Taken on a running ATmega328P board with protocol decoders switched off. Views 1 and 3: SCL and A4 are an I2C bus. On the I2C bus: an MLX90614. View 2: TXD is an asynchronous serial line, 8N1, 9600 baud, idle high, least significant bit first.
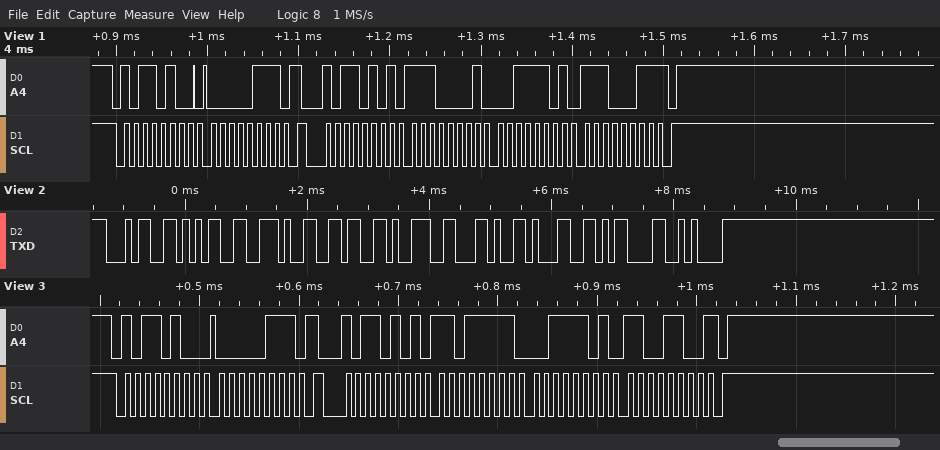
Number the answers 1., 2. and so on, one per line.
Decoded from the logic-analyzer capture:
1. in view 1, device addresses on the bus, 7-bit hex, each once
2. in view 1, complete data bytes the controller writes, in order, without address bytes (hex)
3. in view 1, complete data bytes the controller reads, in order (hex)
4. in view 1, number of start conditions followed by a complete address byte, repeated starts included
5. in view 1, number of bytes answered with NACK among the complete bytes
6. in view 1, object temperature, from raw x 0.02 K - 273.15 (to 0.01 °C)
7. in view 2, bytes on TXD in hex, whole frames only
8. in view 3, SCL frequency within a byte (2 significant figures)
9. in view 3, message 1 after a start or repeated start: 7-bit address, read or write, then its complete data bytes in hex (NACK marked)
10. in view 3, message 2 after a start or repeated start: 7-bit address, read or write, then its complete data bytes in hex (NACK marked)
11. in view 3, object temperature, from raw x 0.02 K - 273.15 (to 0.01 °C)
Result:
1. 0x5A
2. 07
3. E1 3D E3
4. 2
5. 1
6. 43.67 °C
7. 0x34 0x35 0x2E 0x36 0x39 0x2C 0x31 0x0D 0x0A
8. 100 kHz
9. 0x5A write: 07
10. 0x5A read: DF 3D CC NACK
11. 43.63 °C
